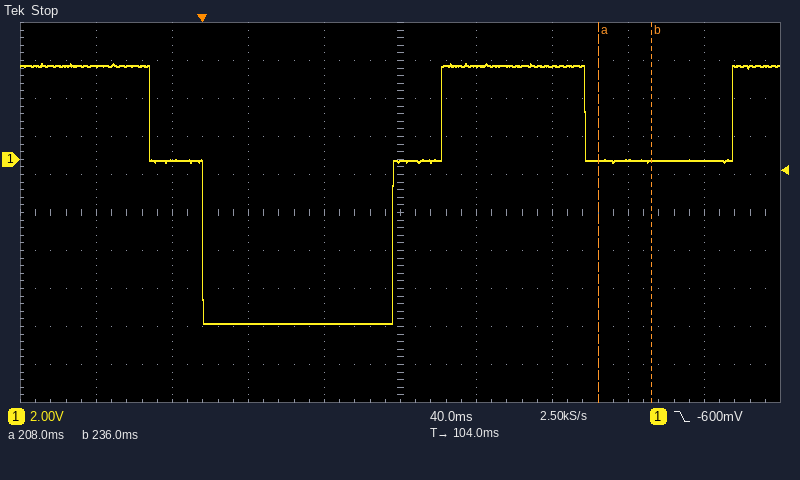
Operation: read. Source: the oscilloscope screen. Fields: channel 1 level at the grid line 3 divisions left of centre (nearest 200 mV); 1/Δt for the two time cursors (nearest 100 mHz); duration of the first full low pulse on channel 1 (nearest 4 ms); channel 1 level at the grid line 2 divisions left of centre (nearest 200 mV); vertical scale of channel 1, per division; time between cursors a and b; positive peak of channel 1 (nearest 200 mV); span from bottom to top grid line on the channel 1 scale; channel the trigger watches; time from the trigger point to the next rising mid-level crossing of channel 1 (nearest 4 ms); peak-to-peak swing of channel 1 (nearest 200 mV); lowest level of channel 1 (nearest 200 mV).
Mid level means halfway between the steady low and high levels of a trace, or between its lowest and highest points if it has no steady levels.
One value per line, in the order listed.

0.0 V
35.7 Hz
100 ms
-8.6 V
2 V
28 ms
5.0 V
20 V
channel 1
100 ms
13.6 V
-8.6 V
